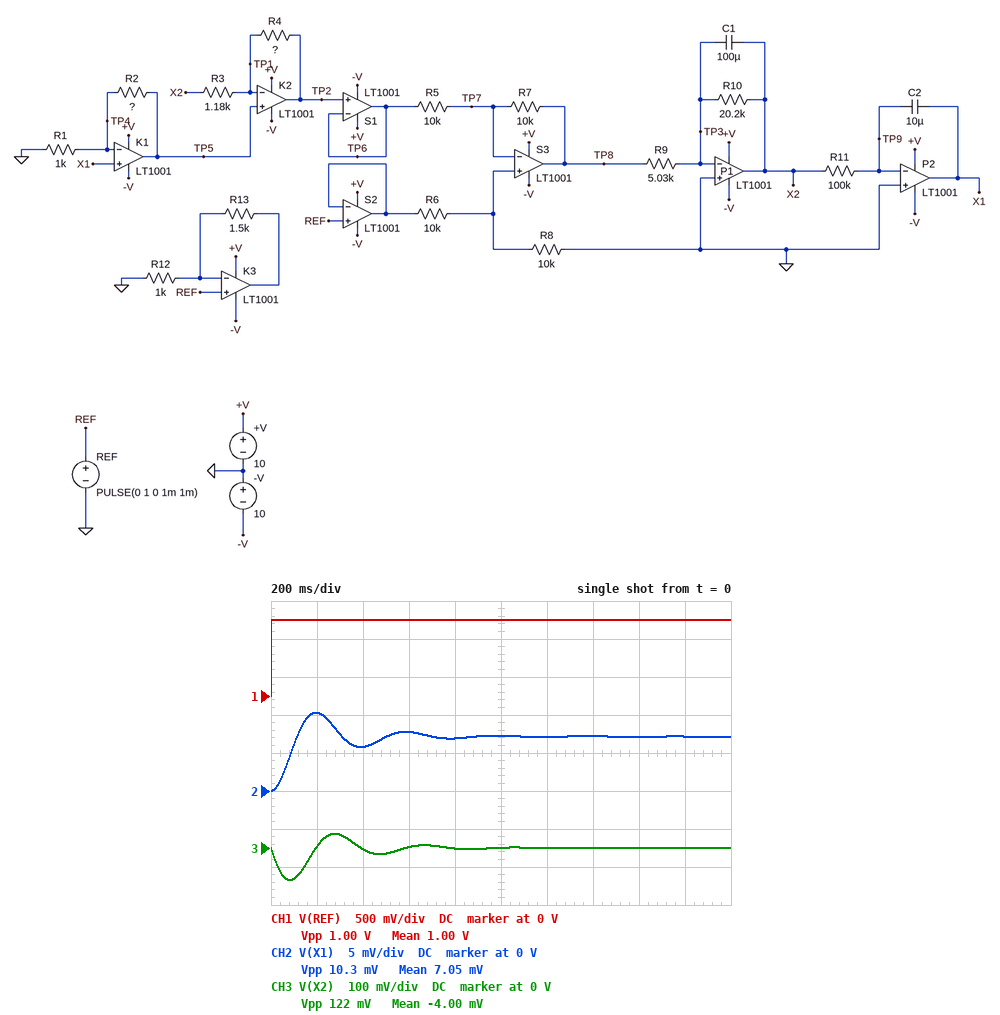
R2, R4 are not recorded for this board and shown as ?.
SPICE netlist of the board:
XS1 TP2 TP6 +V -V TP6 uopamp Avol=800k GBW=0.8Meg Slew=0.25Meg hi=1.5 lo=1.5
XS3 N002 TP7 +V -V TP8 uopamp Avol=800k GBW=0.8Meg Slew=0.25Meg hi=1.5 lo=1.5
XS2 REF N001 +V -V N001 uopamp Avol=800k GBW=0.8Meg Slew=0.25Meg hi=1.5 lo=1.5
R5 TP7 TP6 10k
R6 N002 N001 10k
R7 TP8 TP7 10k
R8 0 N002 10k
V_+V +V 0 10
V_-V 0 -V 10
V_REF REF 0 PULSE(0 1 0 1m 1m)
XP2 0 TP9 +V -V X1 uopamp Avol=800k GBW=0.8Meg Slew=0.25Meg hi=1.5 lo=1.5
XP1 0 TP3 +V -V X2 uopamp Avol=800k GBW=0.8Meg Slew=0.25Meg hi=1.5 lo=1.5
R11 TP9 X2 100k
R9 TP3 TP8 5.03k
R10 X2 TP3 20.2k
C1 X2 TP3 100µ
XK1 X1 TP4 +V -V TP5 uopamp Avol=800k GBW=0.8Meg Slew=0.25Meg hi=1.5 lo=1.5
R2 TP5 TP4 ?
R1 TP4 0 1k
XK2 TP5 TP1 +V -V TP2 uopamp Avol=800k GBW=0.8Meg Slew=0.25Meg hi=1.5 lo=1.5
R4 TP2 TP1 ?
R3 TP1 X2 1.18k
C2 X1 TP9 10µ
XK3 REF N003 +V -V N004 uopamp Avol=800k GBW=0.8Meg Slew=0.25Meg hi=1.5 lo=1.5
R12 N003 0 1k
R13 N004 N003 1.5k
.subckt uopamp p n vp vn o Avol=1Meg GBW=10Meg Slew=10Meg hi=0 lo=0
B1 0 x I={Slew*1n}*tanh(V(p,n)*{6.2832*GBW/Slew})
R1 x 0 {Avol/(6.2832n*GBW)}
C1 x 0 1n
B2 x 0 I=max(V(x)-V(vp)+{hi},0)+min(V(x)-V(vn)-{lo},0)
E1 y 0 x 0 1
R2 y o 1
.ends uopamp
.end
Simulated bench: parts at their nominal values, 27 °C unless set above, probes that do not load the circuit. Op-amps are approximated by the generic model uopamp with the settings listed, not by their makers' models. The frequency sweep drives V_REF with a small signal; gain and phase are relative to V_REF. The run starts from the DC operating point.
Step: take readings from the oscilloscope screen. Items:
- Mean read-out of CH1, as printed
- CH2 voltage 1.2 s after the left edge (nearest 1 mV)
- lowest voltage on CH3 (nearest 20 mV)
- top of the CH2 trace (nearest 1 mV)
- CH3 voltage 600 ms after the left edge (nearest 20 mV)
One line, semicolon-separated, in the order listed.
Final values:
1.00 V; 7 mV; -80 mV; 10 mV; 0 V
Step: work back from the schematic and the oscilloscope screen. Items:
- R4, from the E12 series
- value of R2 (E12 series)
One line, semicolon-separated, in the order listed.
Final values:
4.7 kΩ; 27 kΩ
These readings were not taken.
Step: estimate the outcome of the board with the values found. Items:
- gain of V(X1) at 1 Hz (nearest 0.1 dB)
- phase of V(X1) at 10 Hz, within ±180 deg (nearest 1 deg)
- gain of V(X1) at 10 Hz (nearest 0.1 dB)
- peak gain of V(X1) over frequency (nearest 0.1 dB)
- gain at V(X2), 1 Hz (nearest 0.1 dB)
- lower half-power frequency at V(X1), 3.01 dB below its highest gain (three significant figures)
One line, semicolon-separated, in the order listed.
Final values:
-41.8 dB; -172 deg; -65.4 dB; -36.7 dB; -25.8 dB; 1.64 Hz
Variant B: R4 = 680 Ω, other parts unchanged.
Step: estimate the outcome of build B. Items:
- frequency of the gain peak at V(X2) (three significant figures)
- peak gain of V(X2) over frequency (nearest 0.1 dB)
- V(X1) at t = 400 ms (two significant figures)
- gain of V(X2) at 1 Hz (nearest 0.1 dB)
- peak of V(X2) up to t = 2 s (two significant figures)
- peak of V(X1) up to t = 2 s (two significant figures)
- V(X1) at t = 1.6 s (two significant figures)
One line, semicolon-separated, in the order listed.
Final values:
1.49 Hz; 1.7 dB; 37 mV; -11.9 dB; 140 mV; 40 mV; 27 mV
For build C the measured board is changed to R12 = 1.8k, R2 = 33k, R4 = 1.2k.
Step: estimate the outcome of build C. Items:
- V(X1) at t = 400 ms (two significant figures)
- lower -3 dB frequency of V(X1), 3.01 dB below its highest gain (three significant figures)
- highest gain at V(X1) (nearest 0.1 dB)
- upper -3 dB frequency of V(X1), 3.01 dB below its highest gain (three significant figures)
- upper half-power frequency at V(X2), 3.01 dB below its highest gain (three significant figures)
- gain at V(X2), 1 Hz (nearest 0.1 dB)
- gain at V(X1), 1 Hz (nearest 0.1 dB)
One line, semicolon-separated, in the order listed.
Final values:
16 mV; 1.62 Hz; -23.3 dB; 2.03 Hz; 2.07 Hz; -17.9 dB; -33.9 dB
